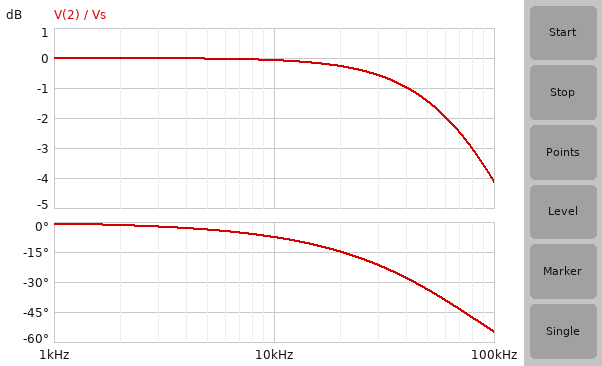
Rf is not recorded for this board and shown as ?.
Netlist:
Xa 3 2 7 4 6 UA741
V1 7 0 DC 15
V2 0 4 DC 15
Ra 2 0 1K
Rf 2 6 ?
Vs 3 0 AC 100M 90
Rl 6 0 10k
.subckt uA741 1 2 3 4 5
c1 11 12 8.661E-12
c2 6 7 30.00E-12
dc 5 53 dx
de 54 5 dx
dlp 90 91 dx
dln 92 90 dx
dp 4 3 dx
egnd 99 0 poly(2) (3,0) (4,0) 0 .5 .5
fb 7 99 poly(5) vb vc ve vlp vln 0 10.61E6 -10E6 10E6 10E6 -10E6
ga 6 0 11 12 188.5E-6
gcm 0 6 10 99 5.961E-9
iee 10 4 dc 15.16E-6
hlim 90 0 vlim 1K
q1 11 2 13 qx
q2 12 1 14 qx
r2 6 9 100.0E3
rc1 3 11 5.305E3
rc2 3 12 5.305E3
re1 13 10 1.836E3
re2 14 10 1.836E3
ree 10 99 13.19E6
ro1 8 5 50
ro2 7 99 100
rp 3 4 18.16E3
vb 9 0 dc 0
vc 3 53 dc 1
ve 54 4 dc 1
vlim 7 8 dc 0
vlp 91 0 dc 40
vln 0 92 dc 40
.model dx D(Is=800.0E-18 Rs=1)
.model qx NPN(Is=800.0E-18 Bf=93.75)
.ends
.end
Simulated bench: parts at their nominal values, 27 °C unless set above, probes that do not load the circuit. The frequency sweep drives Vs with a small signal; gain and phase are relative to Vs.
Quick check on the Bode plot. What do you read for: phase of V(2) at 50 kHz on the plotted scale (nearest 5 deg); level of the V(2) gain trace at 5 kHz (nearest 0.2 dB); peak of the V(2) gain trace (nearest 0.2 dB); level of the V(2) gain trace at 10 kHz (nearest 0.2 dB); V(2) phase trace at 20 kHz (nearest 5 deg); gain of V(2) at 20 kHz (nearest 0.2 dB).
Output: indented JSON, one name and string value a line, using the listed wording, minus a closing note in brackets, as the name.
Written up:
{
  "phase of V(2) at 50 kHz on the plotted scale": "-35 deg",
  "level of the V(2) gain trace at 5 kHz": "0 dB",
  "peak of the V(2) gain trace": "0 dB",
  "level of the V(2) gain trace at 10 kHz": "0 dB",
  "V(2) phase trace at 20 kHz": "-15 deg",
  "gain of V(2) at 20 kHz": "-0.2 dB"
}
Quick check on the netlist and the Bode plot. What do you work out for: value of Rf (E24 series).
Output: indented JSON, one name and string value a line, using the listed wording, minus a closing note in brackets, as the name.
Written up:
{
  "value of Rf": "12 kΩ"
}
